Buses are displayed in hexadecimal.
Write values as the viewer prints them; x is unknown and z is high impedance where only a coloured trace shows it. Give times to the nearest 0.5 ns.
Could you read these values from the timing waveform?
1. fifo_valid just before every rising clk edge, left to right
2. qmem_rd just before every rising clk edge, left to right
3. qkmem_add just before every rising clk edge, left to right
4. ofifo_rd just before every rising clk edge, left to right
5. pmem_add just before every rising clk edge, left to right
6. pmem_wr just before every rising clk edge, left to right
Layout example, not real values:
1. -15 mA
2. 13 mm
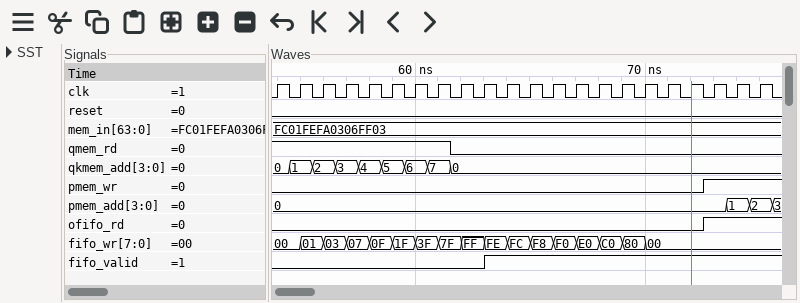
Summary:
1. 0 0 0 0 0 0 0 0 0 0 1 1 1 1 1 1 1 1 1 1 1 1
2. 1 1 1 1 1 1 1 1 0 0 0 0 0 0 0 0 0 0 0 0 0 0
3. 0, 1, 2, 3, 4, 5, 6, 7, 0, 0, 0, 0, 0, 0, 0, 0, 0, 0, 0, 0, 0, 0
4. 0 0 0 0 0 0 0 0 0 0 0 0 0 0 0 0 0 0 0 1 1 1
5. 0, 0, 0, 0, 0, 0, 0, 0, 0, 0, 0, 0, 0, 0, 0, 0, 0, 0, 0, 0, 1, 2
6. 0 0 0 0 0 0 0 0 0 0 0 0 0 0 0 0 0 0 0 1 1 1
